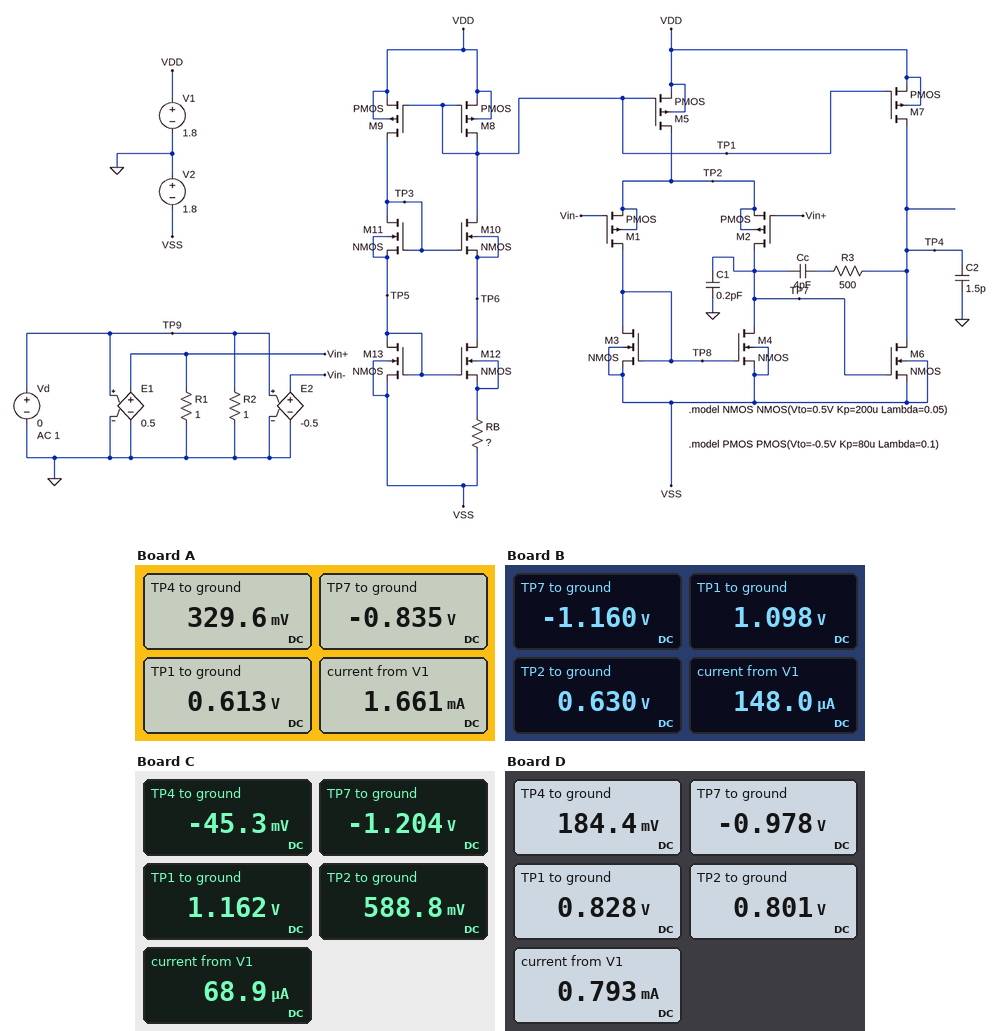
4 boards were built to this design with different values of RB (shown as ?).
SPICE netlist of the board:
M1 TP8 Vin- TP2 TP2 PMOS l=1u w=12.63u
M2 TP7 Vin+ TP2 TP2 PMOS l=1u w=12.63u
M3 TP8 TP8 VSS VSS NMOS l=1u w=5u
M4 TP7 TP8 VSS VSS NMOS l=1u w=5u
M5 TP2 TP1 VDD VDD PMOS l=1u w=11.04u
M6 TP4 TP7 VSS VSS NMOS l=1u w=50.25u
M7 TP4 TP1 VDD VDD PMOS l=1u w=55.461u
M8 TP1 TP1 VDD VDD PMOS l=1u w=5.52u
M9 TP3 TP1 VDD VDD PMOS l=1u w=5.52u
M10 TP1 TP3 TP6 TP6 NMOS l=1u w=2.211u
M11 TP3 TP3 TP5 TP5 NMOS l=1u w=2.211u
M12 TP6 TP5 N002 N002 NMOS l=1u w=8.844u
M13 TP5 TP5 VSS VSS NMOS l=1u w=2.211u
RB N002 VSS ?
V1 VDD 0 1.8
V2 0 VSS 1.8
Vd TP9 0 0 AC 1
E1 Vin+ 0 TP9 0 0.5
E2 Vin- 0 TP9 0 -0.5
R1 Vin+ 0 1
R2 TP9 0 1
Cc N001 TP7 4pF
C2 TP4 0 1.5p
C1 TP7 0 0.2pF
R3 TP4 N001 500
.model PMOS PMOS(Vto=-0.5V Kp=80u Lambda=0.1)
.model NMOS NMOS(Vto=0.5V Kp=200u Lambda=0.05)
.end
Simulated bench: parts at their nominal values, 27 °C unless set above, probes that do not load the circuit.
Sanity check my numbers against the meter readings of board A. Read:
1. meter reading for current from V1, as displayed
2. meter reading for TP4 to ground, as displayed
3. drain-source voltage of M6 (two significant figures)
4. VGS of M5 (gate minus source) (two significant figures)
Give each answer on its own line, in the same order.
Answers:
1.661 mA
329.6 mV
2.1 V
-1.2 V
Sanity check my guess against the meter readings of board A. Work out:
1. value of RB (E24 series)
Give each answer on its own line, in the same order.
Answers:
3 kΩ
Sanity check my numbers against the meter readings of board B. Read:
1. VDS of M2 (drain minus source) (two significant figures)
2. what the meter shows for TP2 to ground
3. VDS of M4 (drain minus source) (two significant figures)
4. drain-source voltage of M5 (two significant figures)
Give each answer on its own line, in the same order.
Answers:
-1.8 V
0.630 V
640 mV
-1.2 V
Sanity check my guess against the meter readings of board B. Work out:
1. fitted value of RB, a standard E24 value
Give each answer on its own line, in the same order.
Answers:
12 kΩ
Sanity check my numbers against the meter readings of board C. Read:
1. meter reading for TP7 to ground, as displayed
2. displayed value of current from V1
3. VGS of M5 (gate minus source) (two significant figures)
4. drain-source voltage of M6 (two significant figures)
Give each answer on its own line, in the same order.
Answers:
-1.204 V
68.9 µA
-640 mV
1.8 V
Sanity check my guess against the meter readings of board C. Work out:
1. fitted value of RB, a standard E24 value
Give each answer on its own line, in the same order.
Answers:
18 kΩ
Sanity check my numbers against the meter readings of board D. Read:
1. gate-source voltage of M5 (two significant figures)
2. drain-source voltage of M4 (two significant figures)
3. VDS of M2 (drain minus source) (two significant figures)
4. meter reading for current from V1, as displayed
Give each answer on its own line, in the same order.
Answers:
-970 mV
820 mV
-1.8 V
0.793 mA
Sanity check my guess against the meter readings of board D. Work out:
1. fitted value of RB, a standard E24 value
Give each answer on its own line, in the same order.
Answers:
4.7 kΩ
